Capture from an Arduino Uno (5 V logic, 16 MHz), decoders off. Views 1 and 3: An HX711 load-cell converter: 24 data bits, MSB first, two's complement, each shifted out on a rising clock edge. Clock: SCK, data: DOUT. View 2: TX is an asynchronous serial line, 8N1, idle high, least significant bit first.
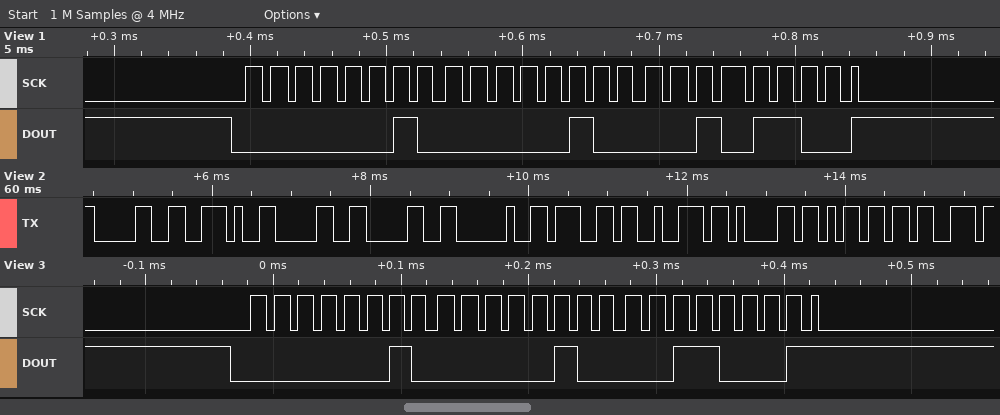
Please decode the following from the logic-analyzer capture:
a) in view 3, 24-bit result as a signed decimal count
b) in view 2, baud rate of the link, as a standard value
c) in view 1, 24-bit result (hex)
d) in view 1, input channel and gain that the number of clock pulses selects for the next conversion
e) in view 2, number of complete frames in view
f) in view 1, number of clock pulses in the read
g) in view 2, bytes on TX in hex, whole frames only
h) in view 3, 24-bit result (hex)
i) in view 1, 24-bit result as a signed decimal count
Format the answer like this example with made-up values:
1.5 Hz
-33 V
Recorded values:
132145
9600 baud
0x02042C
channel A, gain 128
10
25
30 2E 30 30 20 67 72 61 6D 73
0x020431
132140
